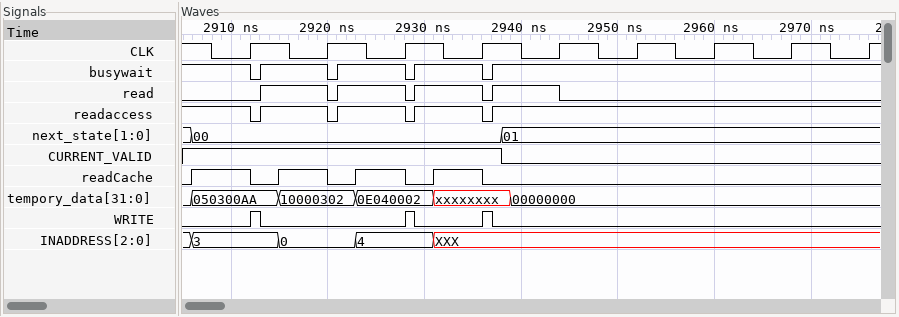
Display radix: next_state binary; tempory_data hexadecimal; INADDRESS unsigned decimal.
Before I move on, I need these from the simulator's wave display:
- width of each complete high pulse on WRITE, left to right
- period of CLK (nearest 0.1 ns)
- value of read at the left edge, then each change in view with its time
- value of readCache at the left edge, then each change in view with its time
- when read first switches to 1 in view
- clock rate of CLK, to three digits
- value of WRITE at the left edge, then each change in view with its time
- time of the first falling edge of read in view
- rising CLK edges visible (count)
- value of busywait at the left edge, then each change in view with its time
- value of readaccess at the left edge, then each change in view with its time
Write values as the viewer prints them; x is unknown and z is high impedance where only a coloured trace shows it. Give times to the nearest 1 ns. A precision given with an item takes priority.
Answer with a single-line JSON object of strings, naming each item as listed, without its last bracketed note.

{"width of each complete high pulse on WRITE, left to right": "1 ns, 1 ns, 1 ns", "period of CLK": "8 ns", "value of read at the left edge, then each change in view with its time": "0, 1 at 2913 ns, 0 at 2920 ns, 1 at 2921 ns, 0 at 2928 ns, 1 at 2929 ns, 0 at 2936 ns, 1 at 2937 ns, 0 at 2944 ns", "value of readCache at the left edge, then each change in view with its time": "0, 1 at 2906 ns, 0 at 2912 ns, 1 at 2915 ns, 0 at 2920 ns, 1 at 2923 ns, 0 at 2928 ns, 1 at 2931 ns, 0 at 2936 ns", "when read first switches to 1 in view": "2913 ns", "clock rate of CLK, to three digits": "125 MHz", "value of WRITE at the left edge, then each change in view with its time": "0, 1 at 2912 ns, 0 at 2913 ns, 1 at 2928 ns, 0 at 2929 ns, 1 at 2936 ns, 0 at 2937 ns", "time of the first falling edge of read in view": "2920 ns", "rising CLK edges visible": "9", "value of busywait at the left edge, then each change in view with its time": "1, 0 at 2912 ns, 1 at 2913 ns, 0 at 2920 ns, 1 at 2921 ns, 0 at 2928 ns, 1 at 2929 ns, 0 at 2936 ns, 1 at 2937 ns", "value of readaccess at the left edge, then each change in view with its time": "1, 0 at 2912 ns, 1 at 2913 ns, 0 at 2920 ns, 1 at 2921 ns, 0 at 2928 ns, 1 at 2929 ns, 0 at 2936 ns, 1 at 2937 ns"}
